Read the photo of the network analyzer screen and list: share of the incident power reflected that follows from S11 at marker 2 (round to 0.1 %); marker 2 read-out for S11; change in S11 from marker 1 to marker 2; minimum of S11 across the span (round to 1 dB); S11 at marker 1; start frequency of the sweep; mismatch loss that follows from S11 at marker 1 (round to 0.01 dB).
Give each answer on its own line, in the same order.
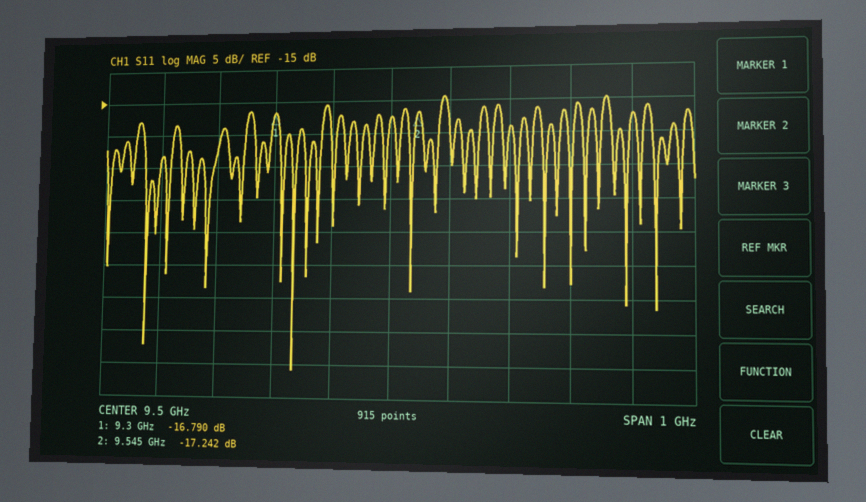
1.9 %
-17.242 dB
-0.452 dB
-56 dB
-16.790 dB
9 GHz
0.09 dB
